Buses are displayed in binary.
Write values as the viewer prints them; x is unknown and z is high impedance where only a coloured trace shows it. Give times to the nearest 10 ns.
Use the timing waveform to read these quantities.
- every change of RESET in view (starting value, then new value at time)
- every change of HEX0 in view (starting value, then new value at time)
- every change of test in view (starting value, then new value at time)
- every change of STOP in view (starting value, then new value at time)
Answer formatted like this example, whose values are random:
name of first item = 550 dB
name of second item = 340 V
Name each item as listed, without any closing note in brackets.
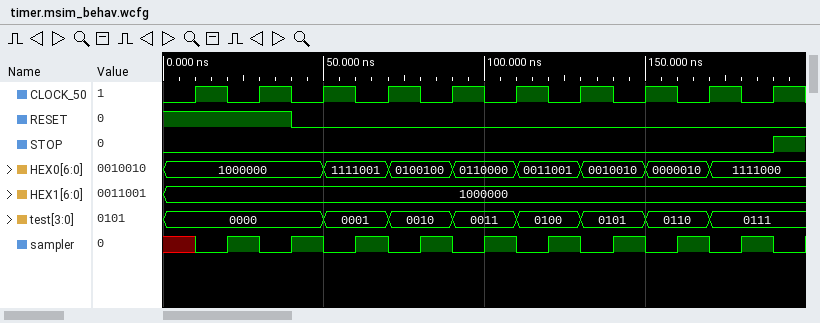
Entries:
every change of RESET in view = 1, 0 at 40 ns
every change of HEX0 in view = 1000000, 1111001 at 50 ns, 0100100 at 70 ns, 0110000 at 90 ns, 0011001 at 110 ns, 0010010 at 130 ns, 0000010 at 150 ns, 1111000 at 170 ns
every change of test in view = 0000, 0001 at 50 ns, 0010 at 70 ns, 0011 at 90 ns, 0100 at 110 ns, 0101 at 130 ns, 0110 at 150 ns, 0111 at 170 ns
every change of STOP in view = 0, 1 at 190 ns
